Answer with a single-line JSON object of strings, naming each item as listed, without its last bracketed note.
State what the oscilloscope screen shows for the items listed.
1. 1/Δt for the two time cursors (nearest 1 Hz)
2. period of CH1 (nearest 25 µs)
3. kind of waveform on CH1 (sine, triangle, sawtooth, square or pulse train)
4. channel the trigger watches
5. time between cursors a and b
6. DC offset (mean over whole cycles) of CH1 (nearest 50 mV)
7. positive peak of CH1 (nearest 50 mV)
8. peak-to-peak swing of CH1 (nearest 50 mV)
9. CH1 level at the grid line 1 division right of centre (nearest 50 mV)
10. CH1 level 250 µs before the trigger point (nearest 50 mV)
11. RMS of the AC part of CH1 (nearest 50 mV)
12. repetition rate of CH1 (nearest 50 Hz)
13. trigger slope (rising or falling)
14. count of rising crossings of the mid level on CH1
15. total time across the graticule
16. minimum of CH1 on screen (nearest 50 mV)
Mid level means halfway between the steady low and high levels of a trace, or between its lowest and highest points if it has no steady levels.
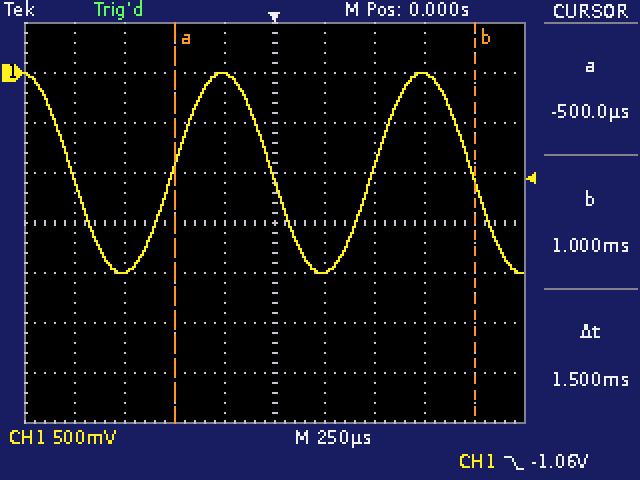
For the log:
{"1/Δt for the two time cursors": "667 Hz", "period of CH1": "1.000 ms", "kind of waveform on CH1": "sine", "channel the trigger watches": "CH1", "time between cursors a and b": "1.5 ms", "DC offset (mean over whole cycles) of CH1": "-1.00 V", "positive peak of CH1": "0 mV", "peak-to-peak swing of CH1": "2.00 V", "CH1 level at the grid line 1 division right of centre": "-2.00 V", "CH1 level 250 µs before the trigger point": "0 mV", "RMS of the AC part of CH1": "700 mV", "repetition rate of CH1": "1.00 kHz", "trigger slope": "falling", "count of rising crossings of the mid level on CH1": "2", "total time across the graticule": "2.5 ms", "minimum of CH1 on screen": "-2.00 V"}
